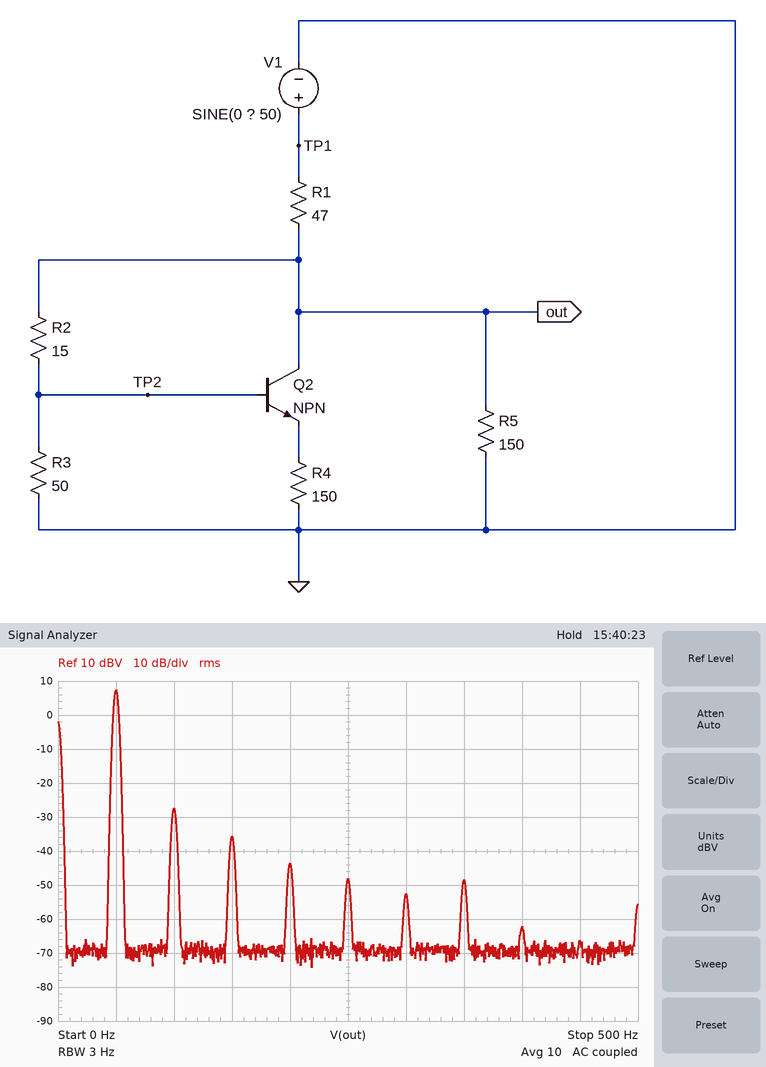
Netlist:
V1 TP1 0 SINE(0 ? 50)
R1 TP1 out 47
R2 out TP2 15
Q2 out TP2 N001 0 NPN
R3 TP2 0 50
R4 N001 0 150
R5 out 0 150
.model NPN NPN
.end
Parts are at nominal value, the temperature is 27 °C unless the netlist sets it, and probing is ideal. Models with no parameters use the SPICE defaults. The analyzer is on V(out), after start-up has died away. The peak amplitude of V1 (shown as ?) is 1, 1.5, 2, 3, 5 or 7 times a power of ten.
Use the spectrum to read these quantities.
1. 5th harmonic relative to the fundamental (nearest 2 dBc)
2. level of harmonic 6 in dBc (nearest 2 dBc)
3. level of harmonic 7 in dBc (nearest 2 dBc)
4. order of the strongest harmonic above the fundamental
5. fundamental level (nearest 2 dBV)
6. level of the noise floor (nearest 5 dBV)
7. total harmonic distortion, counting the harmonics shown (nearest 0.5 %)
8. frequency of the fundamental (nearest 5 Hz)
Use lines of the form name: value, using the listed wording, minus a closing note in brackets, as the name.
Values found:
5th harmonic relative to the fundamental: -56 dBc
level of harmonic 6 in dBc: -60 dBc
level of harmonic 7 in dBc: -56 dBc
order of the strongest harmonic above the fundamental: 2
fundamental level: 8 dBV
level of the noise floor: -70 dBV
total harmonic distortion, counting the harmonics shown: 2.0 %
frequency of the fundamental: 50 Hz
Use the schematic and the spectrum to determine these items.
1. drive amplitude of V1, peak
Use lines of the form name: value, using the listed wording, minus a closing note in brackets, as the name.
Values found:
drive amplitude of V1, peak: 7 V
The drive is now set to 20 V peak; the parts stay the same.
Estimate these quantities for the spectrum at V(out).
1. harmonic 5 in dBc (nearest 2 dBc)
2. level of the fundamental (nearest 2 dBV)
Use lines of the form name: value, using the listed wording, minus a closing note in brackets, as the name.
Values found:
harmonic 5 in dBc: -38 dBc
level of the fundamental: 16 dBV
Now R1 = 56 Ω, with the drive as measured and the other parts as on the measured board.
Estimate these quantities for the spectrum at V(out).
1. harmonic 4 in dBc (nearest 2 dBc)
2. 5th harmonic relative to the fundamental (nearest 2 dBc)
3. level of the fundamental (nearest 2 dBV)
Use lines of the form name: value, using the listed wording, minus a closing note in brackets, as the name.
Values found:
harmonic 4 in dBc: -56 dBc
5th harmonic relative to the fundamental: -52 dBc
level of the fundamental: 6 dBV
